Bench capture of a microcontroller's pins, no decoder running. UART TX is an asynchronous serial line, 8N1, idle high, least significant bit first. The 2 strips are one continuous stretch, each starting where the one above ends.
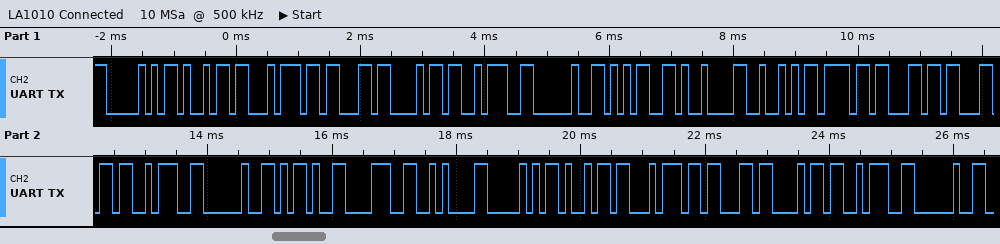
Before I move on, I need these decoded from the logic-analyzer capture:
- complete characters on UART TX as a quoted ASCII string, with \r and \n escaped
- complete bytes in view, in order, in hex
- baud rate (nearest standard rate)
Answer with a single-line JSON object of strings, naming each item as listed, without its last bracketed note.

{"complete characters on UART TX as a quoted ASCII string, with \\r and \\n escaped": "\"Pitch: 5\\tRoll: -8\\nPitch: \"", "complete bytes in view, in order, in hex": "50 69 74 63 68 3A 20 35 09 52 6F 6C 6C 3A 20 2D 38 0A 50 69 74 63 68 3A 20", "baud rate": "9600 baud"}
